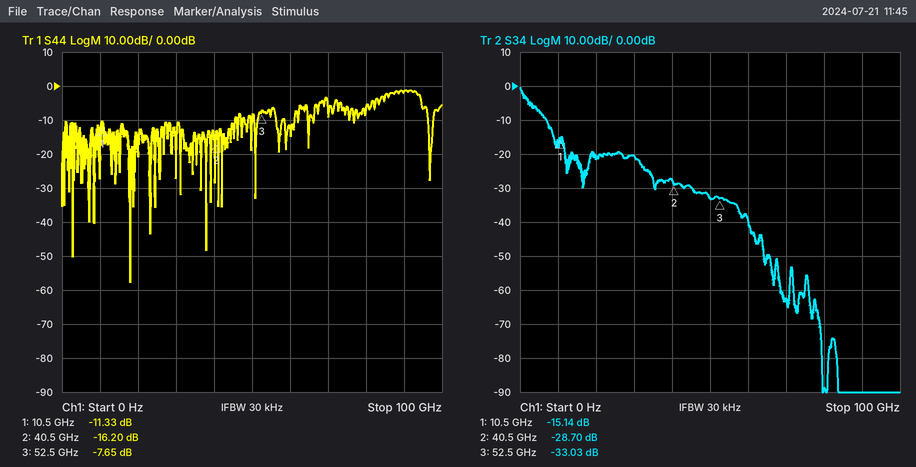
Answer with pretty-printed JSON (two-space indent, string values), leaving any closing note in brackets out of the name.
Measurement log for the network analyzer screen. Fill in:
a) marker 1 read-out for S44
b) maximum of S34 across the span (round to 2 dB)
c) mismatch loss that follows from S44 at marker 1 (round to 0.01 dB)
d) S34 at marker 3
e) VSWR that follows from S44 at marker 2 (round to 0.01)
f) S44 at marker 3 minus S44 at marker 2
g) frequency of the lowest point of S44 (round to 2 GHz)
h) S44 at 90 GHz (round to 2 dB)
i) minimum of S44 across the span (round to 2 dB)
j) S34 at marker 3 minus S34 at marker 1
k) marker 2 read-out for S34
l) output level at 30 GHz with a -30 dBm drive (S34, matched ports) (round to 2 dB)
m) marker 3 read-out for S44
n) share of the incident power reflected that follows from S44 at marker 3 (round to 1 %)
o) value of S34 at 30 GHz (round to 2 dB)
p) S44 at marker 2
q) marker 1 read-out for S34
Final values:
{
  "marker 1 read-out for S44": "-11.33 dB",
  "maximum of S34 across the span": "0 dB",
  "mismatch loss that follows from S44 at marker 1": "0.33 dB",
  "S34 at marker 3": "-33.03 dB",
  "VSWR that follows from S44 at marker 2": "1.37",
  "S44 at marker 3 minus S44 at marker 2": "8.55 dB",
  "frequency of the lowest point of S44": "18 GHz",
  "S44 at 90 GHz": "-2 dB",
  "minimum of S44 across the span": "-58 dB",
  "S34 at marker 3 minus S34 at marker 1": "-17.89 dB",
  "marker 2 read-out for S34": "-28.70 dB",
  "output level at 30 GHz with a -30 dBm drive (S34, matched ports)": "-50 dBm",
  "marker 3 read-out for S44": "-7.65 dB",
  "share of the incident power reflected that follows from S44 at marker 3": "17 %",
  "value of S34 at 30 GHz": "-20 dB",
  "S44 at marker 2": "-16.20 dB",
  "marker 1 read-out for S34": "-15.14 dB"
}
